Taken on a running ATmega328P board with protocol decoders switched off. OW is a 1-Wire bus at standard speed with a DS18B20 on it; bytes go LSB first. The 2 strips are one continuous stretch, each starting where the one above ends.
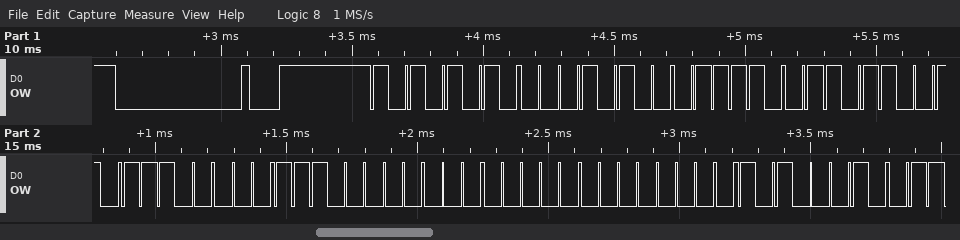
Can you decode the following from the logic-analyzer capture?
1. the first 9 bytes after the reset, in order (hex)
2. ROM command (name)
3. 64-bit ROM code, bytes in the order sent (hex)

55 28 9E 4D 07 07 00 00 45
Match ROM
28 9E 4D 07 07 00 00 45
